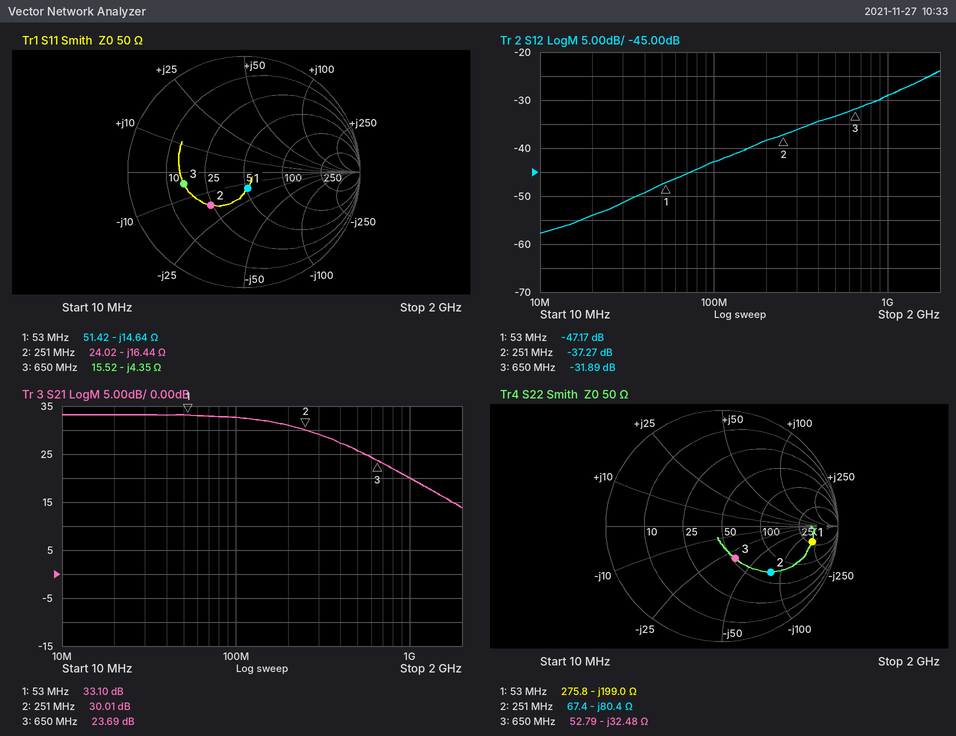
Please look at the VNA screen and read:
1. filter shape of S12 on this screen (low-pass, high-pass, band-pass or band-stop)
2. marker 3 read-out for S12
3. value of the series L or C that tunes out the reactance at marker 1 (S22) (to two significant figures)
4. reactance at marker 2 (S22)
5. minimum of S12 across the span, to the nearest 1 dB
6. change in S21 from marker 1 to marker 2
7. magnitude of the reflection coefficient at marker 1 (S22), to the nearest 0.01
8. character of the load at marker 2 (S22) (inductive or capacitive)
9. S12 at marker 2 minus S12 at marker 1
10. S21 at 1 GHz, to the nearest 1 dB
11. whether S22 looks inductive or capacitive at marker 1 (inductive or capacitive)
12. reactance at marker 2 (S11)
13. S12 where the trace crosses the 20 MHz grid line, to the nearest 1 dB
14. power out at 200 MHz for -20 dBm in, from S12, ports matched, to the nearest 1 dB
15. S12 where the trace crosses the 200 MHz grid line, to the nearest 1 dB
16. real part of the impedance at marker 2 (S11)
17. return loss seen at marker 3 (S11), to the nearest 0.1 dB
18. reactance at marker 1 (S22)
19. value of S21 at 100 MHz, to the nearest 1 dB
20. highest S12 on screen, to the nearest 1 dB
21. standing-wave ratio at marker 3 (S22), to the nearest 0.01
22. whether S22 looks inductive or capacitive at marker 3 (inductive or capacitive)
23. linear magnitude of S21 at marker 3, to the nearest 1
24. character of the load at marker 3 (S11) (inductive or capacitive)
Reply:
high-pass
-31.89 dB
600 nH
-80.4 Ω
-58 dB
-3.09 dB
0.79
capacitive
9.90 dB
20 dB
capacitive
-16.44 Ω
-54 dB
-58 dBm
-38 dB
24.02 Ω
5.5 dB
-199.0 Ω
33 dB
-24 dB
1.87
capacitive
15
capacitive
